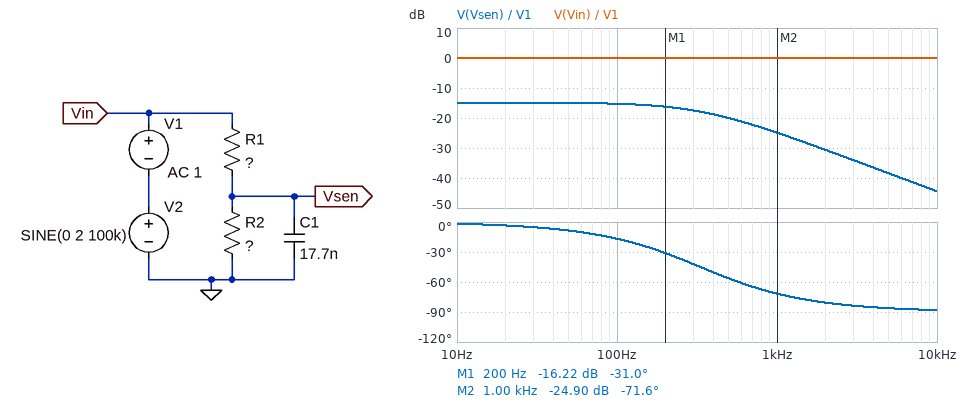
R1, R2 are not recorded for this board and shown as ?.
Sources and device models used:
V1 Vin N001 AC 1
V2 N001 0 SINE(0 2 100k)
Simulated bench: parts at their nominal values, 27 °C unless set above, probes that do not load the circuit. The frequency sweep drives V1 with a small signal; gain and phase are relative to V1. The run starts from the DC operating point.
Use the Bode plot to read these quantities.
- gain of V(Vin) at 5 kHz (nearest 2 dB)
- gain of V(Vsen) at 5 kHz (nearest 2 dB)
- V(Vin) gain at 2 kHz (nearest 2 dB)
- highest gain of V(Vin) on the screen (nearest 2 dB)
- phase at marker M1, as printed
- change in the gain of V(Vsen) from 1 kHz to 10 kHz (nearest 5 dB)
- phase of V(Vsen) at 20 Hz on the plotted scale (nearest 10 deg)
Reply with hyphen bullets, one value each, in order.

- 0 dB
- -38 dB
- 0 dB
- 0 dB
- -31.0 deg
- -20 dB
- 0 deg
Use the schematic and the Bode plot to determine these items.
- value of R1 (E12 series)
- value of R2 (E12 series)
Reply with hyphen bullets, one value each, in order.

- 150 kΩ
- 33 kΩ
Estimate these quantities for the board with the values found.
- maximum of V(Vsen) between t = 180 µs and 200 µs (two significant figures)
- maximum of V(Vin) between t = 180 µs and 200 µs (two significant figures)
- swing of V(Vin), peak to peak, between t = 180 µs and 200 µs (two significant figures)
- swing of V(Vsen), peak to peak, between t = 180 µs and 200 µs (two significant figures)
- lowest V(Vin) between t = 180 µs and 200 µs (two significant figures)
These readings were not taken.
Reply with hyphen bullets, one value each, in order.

- 2.0 mV
- 2.0 V
- 4.0 V
- 2.4 mV
- -2.0 V
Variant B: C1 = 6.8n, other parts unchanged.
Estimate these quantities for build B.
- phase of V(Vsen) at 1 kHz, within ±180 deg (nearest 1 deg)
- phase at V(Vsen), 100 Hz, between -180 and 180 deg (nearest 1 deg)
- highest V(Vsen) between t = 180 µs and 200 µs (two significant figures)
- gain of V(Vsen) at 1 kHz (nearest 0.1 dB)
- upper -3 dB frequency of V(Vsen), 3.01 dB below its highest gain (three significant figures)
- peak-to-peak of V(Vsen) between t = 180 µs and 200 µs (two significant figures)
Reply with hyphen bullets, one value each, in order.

- -49 deg
- -7 deg
- 4.3 mV
- -18.6 dB
- 865 Hz
- 6.3 mV
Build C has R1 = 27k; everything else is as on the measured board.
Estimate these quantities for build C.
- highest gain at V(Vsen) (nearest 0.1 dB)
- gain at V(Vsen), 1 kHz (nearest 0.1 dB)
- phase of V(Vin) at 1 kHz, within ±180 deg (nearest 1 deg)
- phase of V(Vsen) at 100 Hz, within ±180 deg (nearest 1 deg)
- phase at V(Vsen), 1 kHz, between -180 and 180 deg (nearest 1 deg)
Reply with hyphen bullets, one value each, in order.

- -5.2 dB
- -10.9 dB
- 0 deg
- -9 deg
- -59 deg
